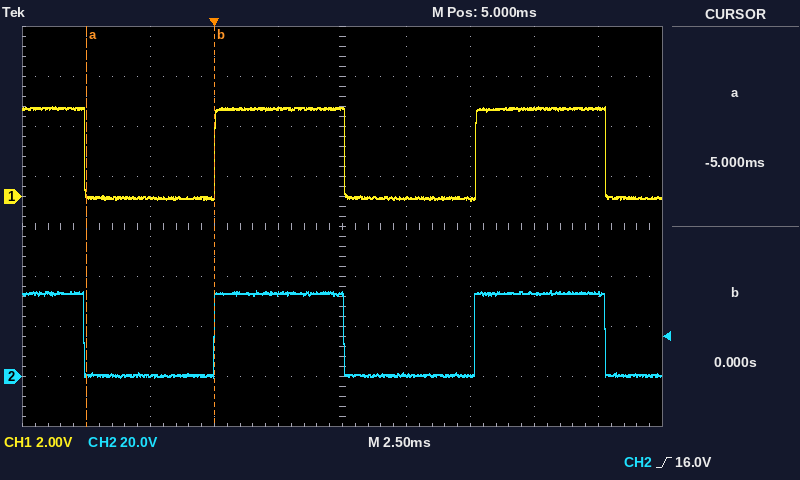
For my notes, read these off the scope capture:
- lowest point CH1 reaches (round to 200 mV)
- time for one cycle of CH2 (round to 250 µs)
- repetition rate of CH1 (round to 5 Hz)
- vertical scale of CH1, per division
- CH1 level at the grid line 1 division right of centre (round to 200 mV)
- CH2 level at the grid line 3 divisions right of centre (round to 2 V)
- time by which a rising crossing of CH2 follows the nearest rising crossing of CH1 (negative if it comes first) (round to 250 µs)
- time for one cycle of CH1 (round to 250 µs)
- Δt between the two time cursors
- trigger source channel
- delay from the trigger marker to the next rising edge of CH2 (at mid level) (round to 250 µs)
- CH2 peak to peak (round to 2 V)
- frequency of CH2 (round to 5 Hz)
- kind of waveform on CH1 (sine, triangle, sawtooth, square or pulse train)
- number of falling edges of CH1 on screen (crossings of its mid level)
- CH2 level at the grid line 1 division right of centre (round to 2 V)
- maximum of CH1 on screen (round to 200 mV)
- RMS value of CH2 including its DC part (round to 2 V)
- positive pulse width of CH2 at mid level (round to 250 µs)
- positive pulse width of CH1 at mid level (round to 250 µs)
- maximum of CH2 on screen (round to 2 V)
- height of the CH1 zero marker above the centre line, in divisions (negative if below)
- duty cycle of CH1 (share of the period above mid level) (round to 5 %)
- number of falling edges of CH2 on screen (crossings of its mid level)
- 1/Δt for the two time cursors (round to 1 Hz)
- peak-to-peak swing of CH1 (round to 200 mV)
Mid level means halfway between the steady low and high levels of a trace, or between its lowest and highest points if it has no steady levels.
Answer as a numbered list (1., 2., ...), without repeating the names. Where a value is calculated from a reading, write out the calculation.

1. -200 mV
2. 10.25 ms
3. 1 / 10.25 ms ≈ 97.6 Hz, so 100 Hz to the nearest 5 Hz
4. 2 V
5. 0.0 V
6. 34 V
7. 0.00 ms
8. 10.25 ms
9. 0 s − (-5 ms) = 5.00 ms
10. CH2
11. 10.25 ms
12. 34 V − (0 V) = 34 V
13. 1 / 10.25 ms ≈ 97.6 Hz, so 100 Hz to the nearest 5 Hz
14. square
15. 3
16. 0 V
17. 3.6 V
18. √(0.5 × (34 V)² + 0.5 × (0 V)²) ≈ 24 V
19. 5.00 ms
20. 5.00 ms
21. 34 V
22. +0.6 div
23. 5.00 ms / 10.25 ms ≈ 48.8 %, so 50 % to the nearest 5 %
24. 3
25. 1 / 5.00 ms ≈ 200 Hz
26. 3.6 V − (-200 mV) = 3.8 V
